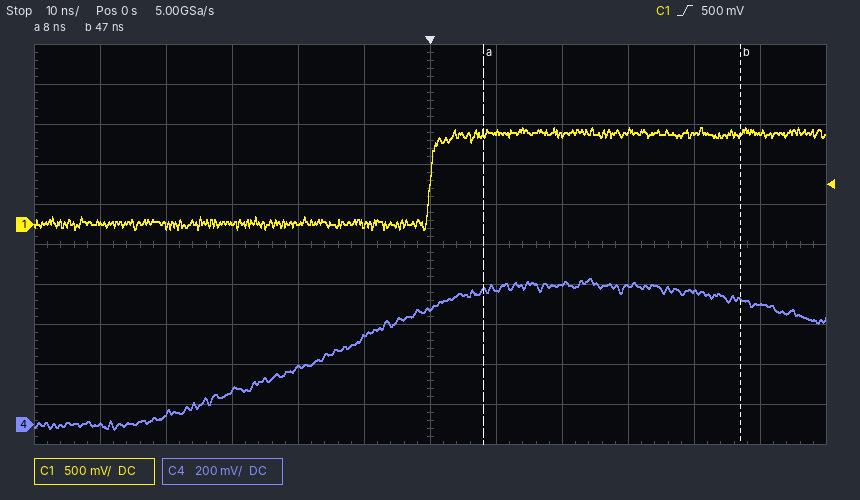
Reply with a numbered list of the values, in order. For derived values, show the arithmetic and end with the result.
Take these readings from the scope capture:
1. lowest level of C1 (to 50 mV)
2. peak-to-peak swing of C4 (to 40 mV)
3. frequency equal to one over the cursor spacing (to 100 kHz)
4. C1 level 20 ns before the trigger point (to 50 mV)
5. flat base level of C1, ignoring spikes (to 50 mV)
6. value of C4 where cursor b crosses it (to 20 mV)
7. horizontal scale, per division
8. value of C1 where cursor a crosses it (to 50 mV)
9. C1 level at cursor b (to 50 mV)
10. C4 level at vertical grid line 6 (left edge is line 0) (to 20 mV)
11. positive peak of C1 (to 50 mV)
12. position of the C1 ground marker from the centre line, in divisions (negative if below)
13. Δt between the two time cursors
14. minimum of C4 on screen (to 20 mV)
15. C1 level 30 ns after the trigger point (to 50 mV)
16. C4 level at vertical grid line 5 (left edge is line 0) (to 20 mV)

1. -50 mV
2. 760 mV
3. 1 / 39 ns ≈ 25.6 MHz
4. 0 mV
5. 0 mV
6. 620 mV
7. 10 ns
8. 1.15 V
9. 1.15 V
10. 580 mV
11. 1.20 V
12. +0.5 div
13. 47 ns − (8 ns) = 39 ns
14. -20 mV
15. 1.15 V
16. 440 mV
